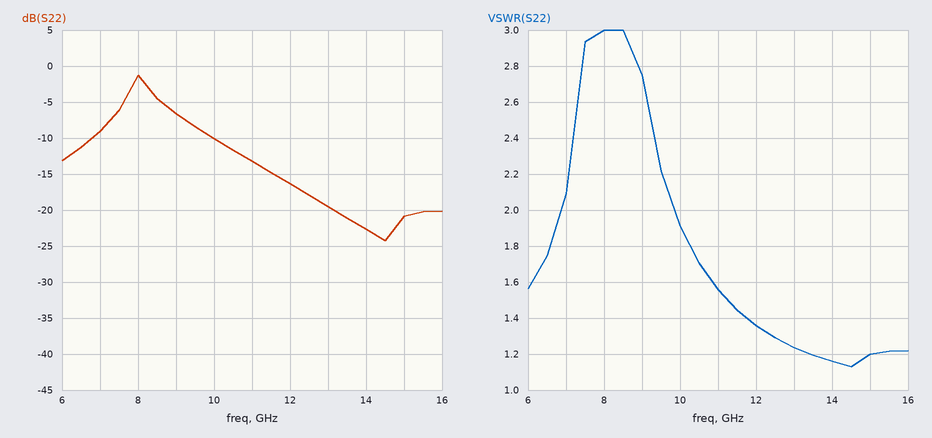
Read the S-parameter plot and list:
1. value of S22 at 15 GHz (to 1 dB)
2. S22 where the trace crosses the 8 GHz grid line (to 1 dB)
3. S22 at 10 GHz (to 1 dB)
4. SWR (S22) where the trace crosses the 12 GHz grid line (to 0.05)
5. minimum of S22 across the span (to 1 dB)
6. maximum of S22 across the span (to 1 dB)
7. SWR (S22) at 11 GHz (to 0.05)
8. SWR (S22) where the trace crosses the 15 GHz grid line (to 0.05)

-21 dB
-1 dB
-10 dB
1.35
-24 dB
-1 dB
1.55
1.20
